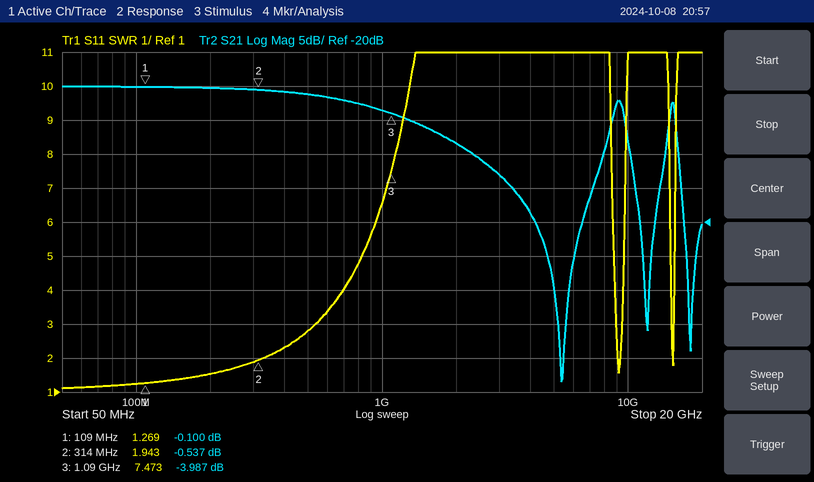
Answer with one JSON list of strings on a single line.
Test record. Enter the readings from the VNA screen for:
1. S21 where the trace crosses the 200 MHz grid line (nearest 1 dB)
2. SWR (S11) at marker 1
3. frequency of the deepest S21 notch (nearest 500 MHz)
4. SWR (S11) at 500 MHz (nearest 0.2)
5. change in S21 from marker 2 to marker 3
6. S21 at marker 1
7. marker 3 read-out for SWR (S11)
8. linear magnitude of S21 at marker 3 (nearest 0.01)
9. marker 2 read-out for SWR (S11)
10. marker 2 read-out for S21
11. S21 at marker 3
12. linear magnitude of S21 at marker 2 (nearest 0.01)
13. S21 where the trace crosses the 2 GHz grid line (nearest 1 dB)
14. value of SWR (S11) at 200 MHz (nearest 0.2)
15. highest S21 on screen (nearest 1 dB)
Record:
["0 dB", "1.269", "5.5 GHz", "2.8", "-3.450 dB", "-0.100 dB", "7.473", "0.63", "1.943", "-0.537 dB", "-3.987 dB", "0.94", "-8 dB", "1.6", "0 dB"]
